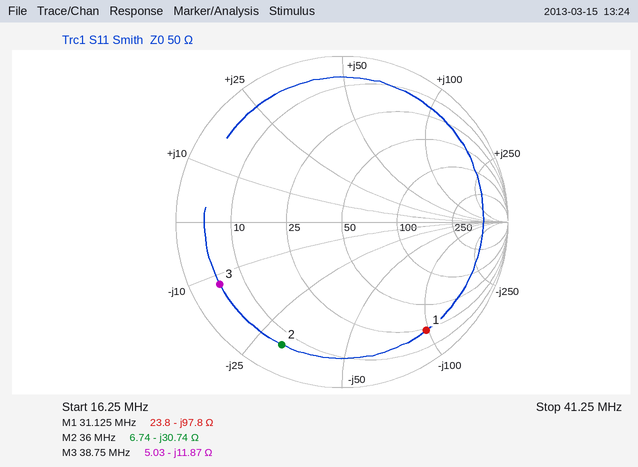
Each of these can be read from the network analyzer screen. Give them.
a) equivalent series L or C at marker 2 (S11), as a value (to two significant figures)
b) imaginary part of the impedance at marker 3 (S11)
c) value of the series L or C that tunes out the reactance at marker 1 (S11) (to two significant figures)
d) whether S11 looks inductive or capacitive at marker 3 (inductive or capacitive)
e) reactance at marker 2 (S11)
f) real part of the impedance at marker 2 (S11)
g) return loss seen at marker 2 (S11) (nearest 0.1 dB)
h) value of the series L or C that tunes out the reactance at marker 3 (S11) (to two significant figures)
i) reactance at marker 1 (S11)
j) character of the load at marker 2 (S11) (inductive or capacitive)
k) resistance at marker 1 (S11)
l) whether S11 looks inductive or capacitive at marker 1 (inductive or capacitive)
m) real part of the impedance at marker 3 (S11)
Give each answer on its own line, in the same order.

140 pF
-11.87 Ω
500 nH
capacitive
-30.74 Ω
6.74 Ω
1.7 dB
49 nH
-97.8 Ω
capacitive
23.8 Ω
capacitive
5.03 Ω
